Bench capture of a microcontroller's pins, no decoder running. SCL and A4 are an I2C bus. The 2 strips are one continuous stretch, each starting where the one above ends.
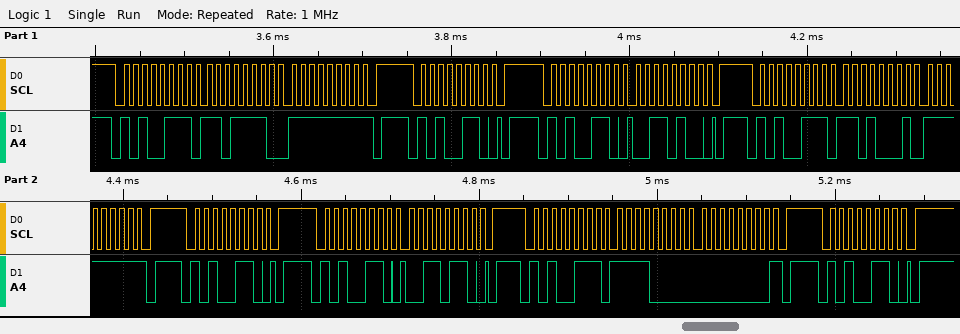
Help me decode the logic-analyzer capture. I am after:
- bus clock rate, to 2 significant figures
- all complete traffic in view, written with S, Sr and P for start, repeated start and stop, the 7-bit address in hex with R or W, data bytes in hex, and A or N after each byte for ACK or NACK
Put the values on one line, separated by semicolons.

100 kHz; S 53R A DE A FF N P S 53W A P S 53W A 34 A P S 53R A D1 A FF N P S 53W A P S 53W A 36 A P S 53R A F0 A 00 N P S 53W A P
